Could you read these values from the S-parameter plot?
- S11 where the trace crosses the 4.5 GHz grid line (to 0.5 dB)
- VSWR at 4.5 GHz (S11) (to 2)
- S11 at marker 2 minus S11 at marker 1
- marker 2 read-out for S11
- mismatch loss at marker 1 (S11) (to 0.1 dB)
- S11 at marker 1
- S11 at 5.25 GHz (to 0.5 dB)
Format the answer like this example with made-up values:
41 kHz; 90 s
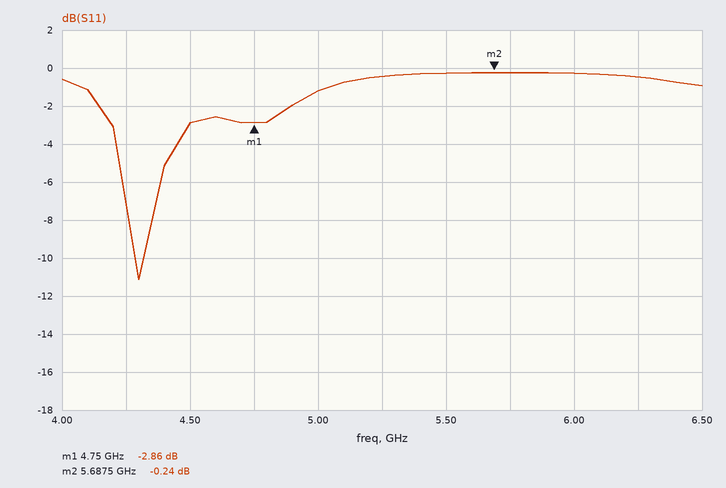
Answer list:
-3.0 dB; 6; 2.62 dB; -0.24 dB; 3.2 dB; -2.86 dB; -0.5 dB
